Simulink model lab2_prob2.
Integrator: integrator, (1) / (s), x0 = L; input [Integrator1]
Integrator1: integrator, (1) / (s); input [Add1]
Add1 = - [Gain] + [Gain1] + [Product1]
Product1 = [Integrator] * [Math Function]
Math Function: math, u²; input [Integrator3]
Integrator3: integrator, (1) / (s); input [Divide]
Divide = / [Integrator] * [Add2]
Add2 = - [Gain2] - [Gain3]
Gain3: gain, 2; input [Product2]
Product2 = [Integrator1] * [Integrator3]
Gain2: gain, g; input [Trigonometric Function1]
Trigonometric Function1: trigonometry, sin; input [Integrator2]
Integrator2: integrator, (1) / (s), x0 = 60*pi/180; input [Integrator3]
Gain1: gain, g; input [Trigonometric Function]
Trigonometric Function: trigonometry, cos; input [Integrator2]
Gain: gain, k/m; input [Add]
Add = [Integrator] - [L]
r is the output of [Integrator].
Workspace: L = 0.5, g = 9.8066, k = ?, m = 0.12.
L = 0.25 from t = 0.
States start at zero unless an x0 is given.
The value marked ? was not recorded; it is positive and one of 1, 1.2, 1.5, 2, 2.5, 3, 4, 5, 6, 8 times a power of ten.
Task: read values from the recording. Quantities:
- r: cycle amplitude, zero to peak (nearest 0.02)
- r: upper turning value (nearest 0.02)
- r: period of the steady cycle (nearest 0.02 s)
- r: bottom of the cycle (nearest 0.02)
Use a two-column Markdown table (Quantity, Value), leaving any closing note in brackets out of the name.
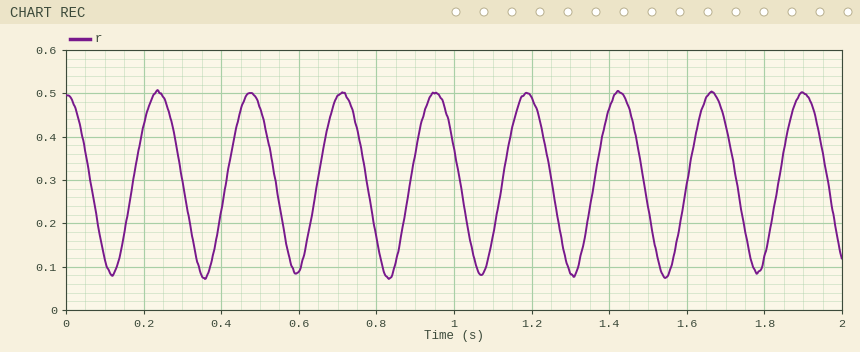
| Quantity | Value |
|---|---|
| r: cycle amplitude, zero to peak | 0.22 |
| r: upper turning value | 0.50 |
| r: period of the steady cycle | 0.24 s |
| r: bottom of the cycle | 0.08 |
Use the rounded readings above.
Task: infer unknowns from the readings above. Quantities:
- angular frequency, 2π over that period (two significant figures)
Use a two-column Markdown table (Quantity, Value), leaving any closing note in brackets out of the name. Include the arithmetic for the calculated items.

| Quantity | Value |
|---|---|
| angular frequency, 2π over that period | 2π / 0.24 = 26 rad/s |
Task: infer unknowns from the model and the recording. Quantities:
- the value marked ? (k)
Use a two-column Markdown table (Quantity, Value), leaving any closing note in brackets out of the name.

| Quantity | Value |
|---|---|
| the value marked ? | 60 |
